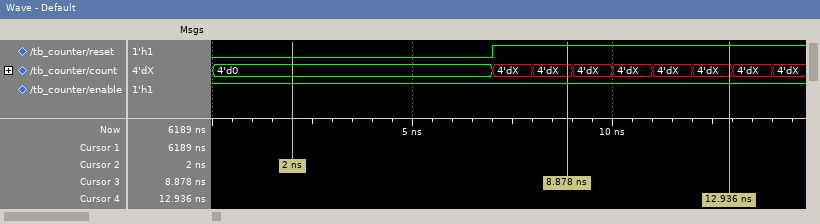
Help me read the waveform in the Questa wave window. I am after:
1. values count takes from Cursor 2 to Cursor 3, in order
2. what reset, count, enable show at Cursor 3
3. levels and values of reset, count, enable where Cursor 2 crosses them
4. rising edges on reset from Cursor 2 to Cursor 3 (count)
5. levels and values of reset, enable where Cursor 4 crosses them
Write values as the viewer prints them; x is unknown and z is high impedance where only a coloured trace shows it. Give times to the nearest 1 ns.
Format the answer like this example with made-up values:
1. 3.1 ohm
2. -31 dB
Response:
1. 4'd0, 4'dX, 4'dX
2. reset=1, count=4'dX, enable=1
3. reset=0, count=4'd0, enable=1
4. 1
5. reset=1, enable=1
